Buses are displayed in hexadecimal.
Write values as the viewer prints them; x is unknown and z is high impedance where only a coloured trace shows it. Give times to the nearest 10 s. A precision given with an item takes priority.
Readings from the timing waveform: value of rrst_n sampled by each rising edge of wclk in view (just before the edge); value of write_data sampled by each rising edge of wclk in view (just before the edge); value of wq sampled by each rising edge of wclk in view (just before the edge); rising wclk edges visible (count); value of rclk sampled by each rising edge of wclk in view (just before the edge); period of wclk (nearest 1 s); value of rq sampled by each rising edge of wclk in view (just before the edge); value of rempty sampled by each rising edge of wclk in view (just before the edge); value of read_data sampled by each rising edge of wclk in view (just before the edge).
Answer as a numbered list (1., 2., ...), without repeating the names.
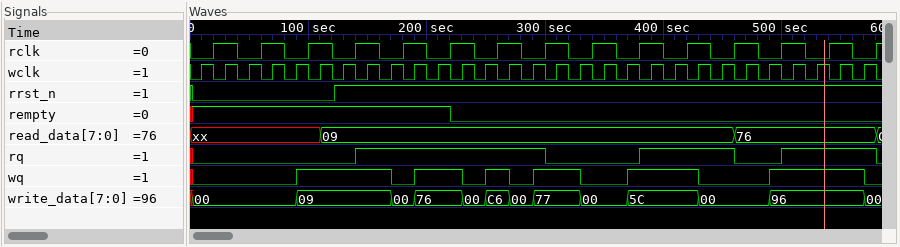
1. 0 0 0 0 0 0 1 1 1 1 1 1 1 1 1 1 1 1 1 1 1 1 1 1 1 1 1 1 1
2. 00, 00, 00, 00, 00, 09, 09, 09, 09, 00, 76, 76, 00, C6, 00, 77, 77, 00, 00, 5C, 5C, 5C, 00, 00, 00, 96, 96, 96, 96
3. 0 0 0 0 0 1 1 1 1 0 1 1 0 1 0 1 1 0 0 1 1 1 0 0 0 1 1 1 1
4. 29
5. 0 1 0 1 0 1 0 1 0 1 0 1 0 1 0 1 0 1 0 1 0 1 0 1 0 1 0 1 0
6. 20 s
7. 0 0 0 0 0 0 0 1 1 1 1 1 1 1 1 0 0 0 0 1 1 1 1 0 0 1 1 1 1
8. 1 1 1 1 1 1 1 1 1 1 1 0 0 0 0 0 0 0 0 0 0 0 0 0 0 0 0 0 0
9. xx, xx, xx, xx, xx, xx, 09, 09, 09, 09, 09, 09, 09, 09, 09, 09, 09, 09, 09, 09, 09, 09, 09, 76, 76, 76, 76, 76, 76
